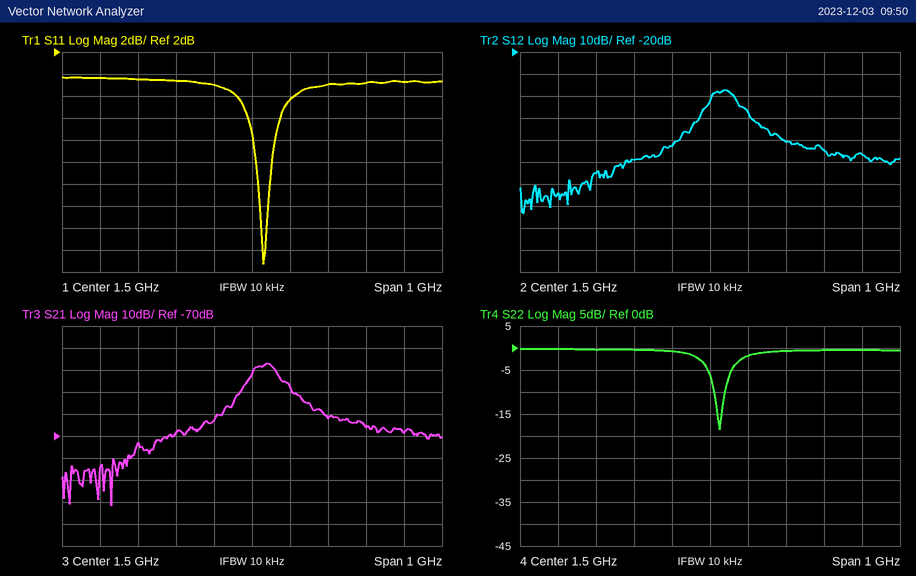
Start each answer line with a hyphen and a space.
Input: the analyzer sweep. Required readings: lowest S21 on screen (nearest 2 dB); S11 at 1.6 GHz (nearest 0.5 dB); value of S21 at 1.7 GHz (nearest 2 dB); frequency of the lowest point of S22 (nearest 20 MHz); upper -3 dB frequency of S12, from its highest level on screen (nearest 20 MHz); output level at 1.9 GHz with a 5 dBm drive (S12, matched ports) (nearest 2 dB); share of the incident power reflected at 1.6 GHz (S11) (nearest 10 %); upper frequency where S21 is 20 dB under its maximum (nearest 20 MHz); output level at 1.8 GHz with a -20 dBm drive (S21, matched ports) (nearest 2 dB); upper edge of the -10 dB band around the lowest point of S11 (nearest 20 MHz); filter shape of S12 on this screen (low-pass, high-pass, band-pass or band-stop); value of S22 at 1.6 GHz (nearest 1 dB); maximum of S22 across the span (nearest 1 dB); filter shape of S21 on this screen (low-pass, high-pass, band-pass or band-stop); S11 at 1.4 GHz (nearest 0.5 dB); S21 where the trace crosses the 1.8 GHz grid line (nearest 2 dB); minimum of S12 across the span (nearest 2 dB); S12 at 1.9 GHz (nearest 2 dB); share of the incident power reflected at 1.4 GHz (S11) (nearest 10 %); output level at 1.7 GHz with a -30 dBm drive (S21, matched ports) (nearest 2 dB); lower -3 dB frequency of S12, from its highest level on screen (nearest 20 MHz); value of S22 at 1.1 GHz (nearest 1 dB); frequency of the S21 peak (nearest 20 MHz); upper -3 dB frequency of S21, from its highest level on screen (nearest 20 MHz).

- -102 dB
- -2.5 dB
- -62 dB
- 1.52 GHz
- 1.56 GHz
- -62 dBm
- 60 %
- 1.66 GHz
- -86 dBm
- 1.54 GHz
- band-pass
- -2 dB
- 0 dB
- band-pass
- -1.0 dB
- -66 dB
- -94 dB
- -66 dB
- 80 %
- -92 dBm
- 1.50 GHz
- 0 dB
- 1.54 GHz
- 1.56 GHz
